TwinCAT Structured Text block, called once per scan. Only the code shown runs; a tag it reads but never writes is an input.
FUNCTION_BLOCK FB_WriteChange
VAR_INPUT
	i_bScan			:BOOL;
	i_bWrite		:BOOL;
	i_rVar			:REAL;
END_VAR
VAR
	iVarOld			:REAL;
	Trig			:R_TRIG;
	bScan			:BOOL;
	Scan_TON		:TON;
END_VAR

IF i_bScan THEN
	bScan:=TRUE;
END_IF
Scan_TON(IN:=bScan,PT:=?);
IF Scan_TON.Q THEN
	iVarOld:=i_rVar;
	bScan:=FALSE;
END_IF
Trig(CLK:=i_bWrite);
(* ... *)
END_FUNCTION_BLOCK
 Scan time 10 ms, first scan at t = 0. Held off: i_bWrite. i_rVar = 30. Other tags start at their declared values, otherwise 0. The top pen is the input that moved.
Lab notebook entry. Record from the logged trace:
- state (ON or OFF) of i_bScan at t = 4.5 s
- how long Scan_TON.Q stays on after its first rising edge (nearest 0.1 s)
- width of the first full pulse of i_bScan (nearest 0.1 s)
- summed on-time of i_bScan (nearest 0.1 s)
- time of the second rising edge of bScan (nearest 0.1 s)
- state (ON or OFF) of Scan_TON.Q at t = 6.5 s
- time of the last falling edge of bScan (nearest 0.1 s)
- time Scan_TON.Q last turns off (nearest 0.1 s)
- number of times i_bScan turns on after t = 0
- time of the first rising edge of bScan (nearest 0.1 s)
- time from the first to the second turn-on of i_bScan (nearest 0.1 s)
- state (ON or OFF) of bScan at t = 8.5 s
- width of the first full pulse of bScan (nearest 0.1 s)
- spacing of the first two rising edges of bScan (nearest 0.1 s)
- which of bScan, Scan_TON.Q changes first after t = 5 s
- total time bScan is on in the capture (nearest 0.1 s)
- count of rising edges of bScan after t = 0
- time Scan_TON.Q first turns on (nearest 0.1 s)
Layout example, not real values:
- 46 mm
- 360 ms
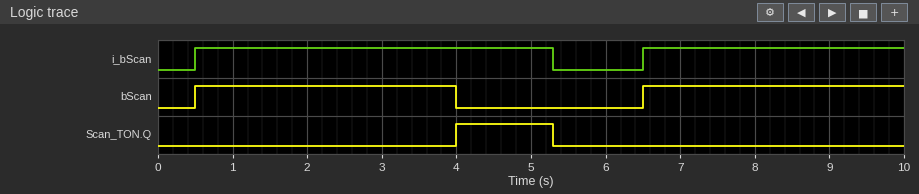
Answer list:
- ON
- 1.3 s
- 4.8 s
- 8.3 s
- 6.5 s
- OFF
- 4.0 s
- 5.3 s
- 2
- 0.5 s
- 6.0 s
- ON
- 3.5 s
- 6.0 s
- Scan_TON.Q
- 7.0 s
- 2
- 4.0 s
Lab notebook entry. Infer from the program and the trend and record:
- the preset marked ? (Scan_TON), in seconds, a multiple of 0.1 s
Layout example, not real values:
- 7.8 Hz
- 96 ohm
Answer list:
- 3.5 s
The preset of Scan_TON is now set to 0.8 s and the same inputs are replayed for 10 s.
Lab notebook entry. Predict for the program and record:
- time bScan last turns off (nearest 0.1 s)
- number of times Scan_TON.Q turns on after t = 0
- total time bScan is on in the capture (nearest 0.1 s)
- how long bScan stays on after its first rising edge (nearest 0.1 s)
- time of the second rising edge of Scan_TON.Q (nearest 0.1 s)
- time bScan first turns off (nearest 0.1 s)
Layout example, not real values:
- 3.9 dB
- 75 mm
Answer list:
- 7.3 s
- 2
- 1.6 s
- 0.8 s
- 7.3 s
- 1.3 s
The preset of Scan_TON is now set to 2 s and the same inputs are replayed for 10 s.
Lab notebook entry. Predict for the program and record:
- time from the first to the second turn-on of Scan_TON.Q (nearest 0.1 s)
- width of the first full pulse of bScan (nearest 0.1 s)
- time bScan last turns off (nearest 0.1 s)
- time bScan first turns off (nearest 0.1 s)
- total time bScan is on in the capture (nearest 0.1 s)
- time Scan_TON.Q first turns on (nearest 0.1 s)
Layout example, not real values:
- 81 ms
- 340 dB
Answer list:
- 6.0 s
- 2.0 s
- 8.5 s
- 2.5 s
- 4.0 s
- 2.5 s
